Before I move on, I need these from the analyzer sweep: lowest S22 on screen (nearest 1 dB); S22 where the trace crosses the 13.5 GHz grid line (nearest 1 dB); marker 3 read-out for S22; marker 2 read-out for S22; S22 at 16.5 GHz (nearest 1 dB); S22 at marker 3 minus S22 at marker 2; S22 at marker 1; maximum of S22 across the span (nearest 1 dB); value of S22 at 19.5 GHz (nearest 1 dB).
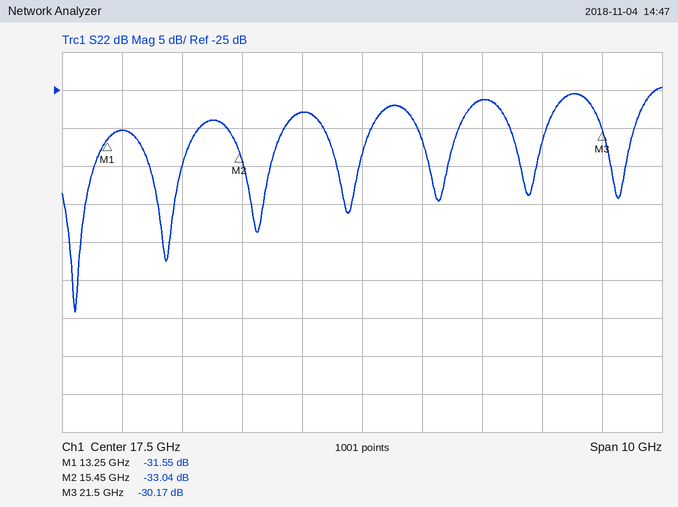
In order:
-54 dB
-30 dB
-30.17 dB
-33.04 dB
-28 dB
2.87 dB
-31.55 dB
-25 dB
-26 dB
